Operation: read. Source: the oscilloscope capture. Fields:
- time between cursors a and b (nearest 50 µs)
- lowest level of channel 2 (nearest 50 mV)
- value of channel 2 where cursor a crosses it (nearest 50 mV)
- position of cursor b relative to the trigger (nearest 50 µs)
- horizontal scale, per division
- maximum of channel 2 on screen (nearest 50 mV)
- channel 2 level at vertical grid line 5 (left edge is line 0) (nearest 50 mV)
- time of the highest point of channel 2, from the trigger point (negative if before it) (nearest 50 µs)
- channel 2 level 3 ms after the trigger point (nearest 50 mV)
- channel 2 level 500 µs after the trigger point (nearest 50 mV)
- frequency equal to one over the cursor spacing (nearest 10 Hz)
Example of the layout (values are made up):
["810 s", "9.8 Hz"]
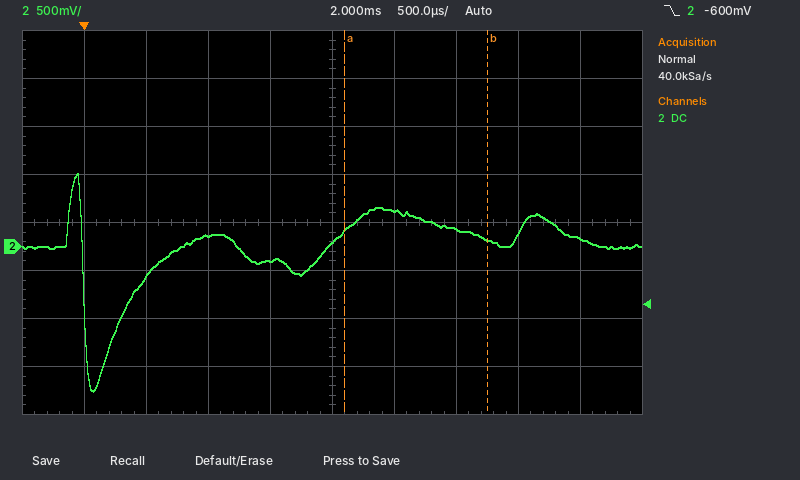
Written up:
["1.15 ms", "-1.50 V", "150 mV", "+3.25 ms", "500 µs", "750 mV", "50 mV", "-50 µs", "200 mV", "-300 mV", "870 Hz"]
